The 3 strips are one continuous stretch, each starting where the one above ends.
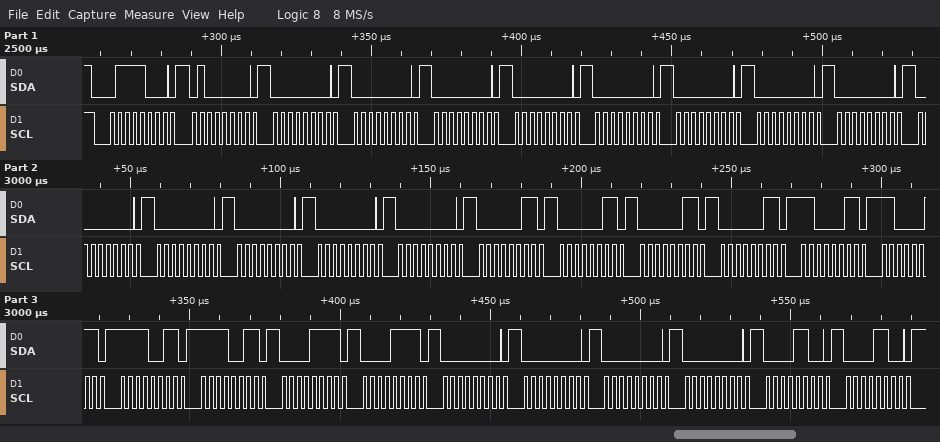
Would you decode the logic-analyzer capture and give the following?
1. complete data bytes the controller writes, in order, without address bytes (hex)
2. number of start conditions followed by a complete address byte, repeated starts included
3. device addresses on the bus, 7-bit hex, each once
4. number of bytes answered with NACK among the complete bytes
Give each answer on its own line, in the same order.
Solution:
40 00 00 00 00 00 00 00 00 00 00 00 00 00 03 03 03 03 C3 C3 F3 F3 0F 0F 00 00 00 00 0C 0C
1
0x3C
0
